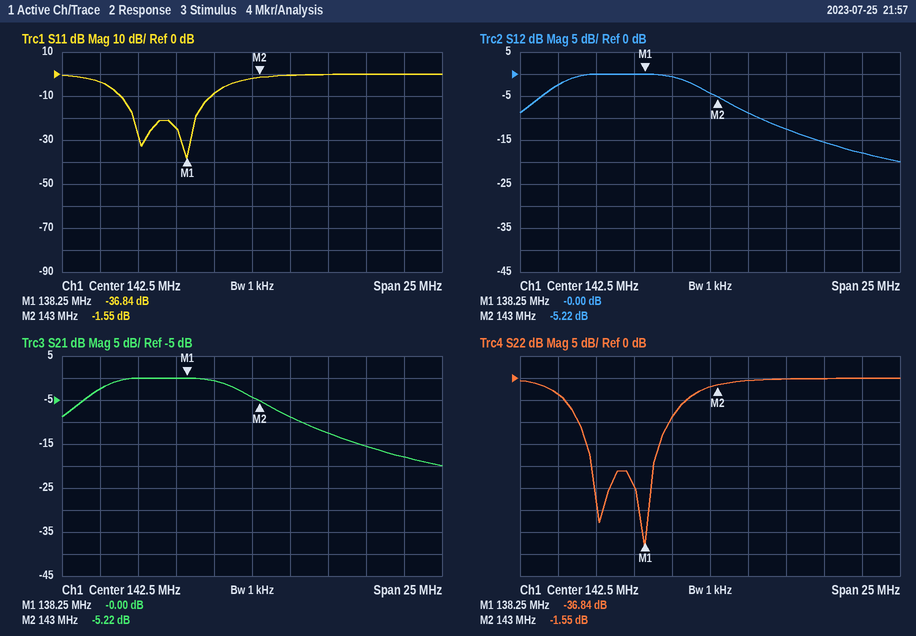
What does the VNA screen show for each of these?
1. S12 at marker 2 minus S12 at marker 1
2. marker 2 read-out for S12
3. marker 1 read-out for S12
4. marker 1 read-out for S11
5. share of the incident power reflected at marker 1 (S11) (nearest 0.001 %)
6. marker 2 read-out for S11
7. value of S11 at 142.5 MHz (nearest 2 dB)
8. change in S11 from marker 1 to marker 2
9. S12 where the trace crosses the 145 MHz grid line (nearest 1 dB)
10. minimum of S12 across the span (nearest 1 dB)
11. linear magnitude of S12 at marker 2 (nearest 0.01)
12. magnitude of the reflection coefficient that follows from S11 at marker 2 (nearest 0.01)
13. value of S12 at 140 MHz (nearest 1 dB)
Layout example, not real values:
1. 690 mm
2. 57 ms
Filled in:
1. -5.22 dB
2. -5.22 dB
3. -0.00 dB
4. -36.84 dB
5. 0.021 %
6. -1.55 dB
7. -2 dB
8. 35.29 dB
9. -9 dB
10. -20 dB
11. 0.55
12. 0.84
13. -1 dB
